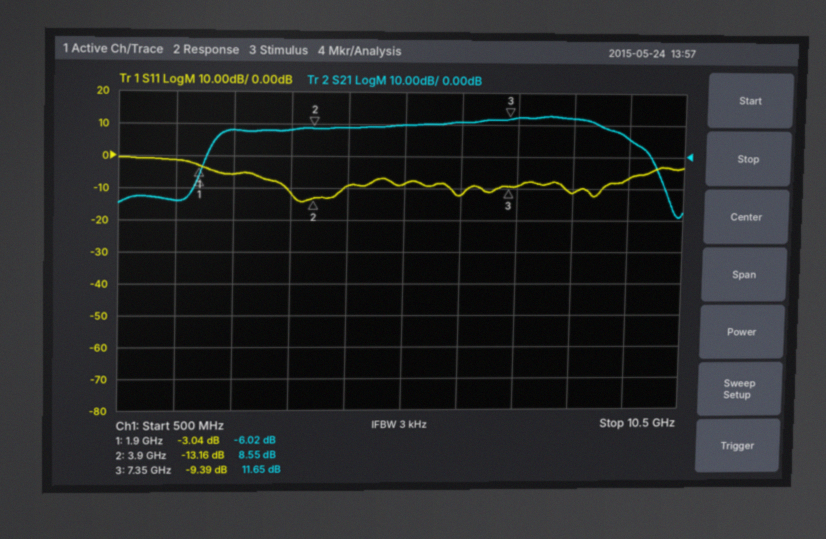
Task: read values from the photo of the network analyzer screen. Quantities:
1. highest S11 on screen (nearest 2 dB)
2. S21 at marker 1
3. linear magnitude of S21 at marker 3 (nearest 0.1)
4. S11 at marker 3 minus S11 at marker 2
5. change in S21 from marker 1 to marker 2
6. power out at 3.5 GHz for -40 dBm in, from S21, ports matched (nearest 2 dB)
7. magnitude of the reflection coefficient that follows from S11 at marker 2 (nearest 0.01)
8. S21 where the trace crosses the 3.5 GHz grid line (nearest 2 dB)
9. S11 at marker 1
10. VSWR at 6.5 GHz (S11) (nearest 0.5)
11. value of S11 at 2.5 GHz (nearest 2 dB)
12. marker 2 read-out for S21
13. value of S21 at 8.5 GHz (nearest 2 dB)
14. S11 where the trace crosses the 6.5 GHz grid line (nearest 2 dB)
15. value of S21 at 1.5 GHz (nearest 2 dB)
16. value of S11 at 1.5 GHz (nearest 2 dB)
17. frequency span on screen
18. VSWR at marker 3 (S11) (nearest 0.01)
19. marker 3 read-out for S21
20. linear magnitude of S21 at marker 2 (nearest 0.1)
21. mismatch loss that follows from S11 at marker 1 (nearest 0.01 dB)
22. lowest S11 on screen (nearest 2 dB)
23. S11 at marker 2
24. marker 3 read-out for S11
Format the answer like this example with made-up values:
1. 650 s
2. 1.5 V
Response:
1. 0 dB
2. -6.02 dB
3. 3.8
4. 3.77 dB
5. 14.57 dB
6. -32 dBm
7. 0.22
8. 8 dB
9. -3.04 dB
10. 1.5
11. -6 dB
12. 8.55 dB
13. 12 dB
14. -12 dB
15. -14 dB
16. -2 dB
17. 10 GHz
18. 2.03
19. 11.65 dB
20. 2.7
21. 2.98 dB
22. -14 dB
23. -13.16 dB
24. -9.39 dB
